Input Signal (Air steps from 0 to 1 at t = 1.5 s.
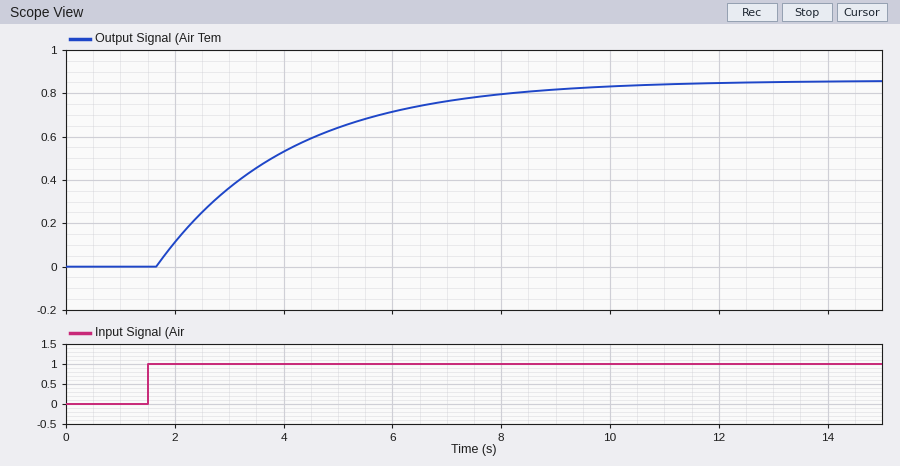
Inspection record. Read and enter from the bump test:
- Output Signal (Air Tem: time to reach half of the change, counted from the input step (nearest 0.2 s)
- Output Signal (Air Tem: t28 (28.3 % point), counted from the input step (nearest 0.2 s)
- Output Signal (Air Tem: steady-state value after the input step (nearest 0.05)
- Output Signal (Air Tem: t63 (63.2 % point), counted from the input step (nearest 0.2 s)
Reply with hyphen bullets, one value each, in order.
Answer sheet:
- 1.8 s
- 1.0 s
- 0.85
- 2.6 s
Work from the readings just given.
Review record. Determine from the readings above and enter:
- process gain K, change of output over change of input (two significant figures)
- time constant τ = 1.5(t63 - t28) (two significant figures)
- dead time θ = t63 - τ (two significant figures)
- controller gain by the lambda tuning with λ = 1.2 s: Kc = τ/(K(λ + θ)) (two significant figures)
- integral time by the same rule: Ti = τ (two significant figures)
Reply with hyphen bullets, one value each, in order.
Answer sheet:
- 0.85
- 2.4 s
- 0.20 s
- 2.0
- 2.4 s
